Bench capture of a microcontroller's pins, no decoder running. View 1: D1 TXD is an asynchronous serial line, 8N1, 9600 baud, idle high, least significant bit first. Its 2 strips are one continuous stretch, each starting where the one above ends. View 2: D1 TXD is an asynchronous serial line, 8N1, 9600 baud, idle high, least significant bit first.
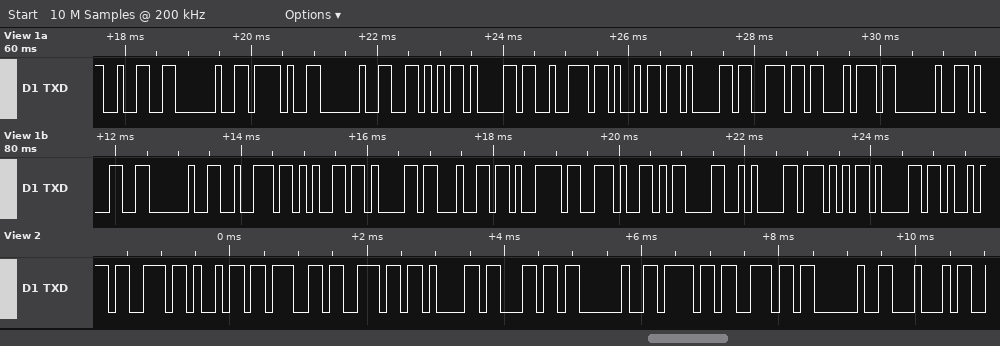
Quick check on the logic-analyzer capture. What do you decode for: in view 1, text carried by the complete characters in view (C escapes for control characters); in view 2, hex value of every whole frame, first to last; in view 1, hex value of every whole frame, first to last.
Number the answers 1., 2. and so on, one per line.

1. "2 / Variant 1 ready.\r\nWa"
2. 0x73 0x69 0x67 0x6E 0x61 0x6C 0x20 0x6F 0x6E 0x20 0x44
3. 32 20 2F 20 56 61 72 69 61 6E 74 20 31 20 72 65 61 64 79 2E 0D 0A 57 61
